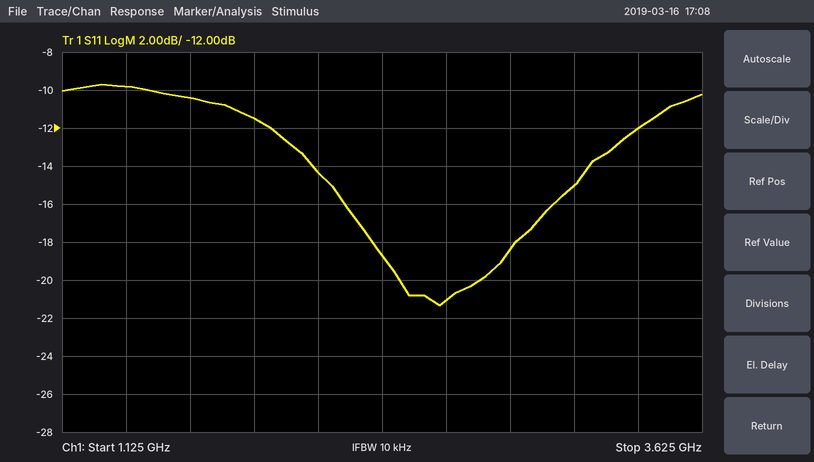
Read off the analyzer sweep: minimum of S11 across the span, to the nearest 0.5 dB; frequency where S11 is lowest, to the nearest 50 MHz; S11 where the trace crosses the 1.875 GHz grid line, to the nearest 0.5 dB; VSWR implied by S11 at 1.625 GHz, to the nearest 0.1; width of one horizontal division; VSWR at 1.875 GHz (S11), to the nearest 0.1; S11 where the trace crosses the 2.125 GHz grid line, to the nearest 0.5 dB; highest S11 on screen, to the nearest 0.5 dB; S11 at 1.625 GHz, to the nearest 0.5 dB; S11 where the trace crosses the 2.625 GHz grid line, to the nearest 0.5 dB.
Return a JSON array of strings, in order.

["-21.5 dB", "2.60 GHz", "-11.5 dB", "1.9", "250 MHz", "1.7", "-14.5 dB", "-9.5 dB", "-10.5 dB", "-21.0 dB"]
